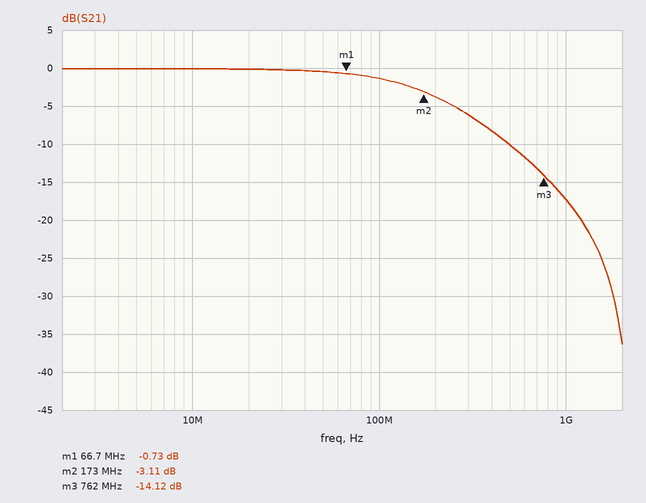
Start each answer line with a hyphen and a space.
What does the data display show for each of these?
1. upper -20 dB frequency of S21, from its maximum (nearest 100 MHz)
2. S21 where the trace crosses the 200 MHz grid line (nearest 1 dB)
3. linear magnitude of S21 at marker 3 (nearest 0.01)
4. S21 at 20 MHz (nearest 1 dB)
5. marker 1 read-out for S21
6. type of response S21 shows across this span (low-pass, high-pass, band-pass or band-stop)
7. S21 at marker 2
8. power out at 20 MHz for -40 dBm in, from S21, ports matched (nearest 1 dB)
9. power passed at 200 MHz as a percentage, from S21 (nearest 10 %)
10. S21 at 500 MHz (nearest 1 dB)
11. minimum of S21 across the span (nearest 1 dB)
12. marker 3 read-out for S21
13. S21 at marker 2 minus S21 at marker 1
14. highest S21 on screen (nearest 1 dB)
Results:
- 1.2 GHz
- -4 dB
- 0.20
- 0 dB
- -0.73 dB
- low-pass
- -3.11 dB
- -40 dBm
- 40 %
- -10 dB
- -36 dB
- -14.12 dB
- -2.38 dB
- 0 dB
